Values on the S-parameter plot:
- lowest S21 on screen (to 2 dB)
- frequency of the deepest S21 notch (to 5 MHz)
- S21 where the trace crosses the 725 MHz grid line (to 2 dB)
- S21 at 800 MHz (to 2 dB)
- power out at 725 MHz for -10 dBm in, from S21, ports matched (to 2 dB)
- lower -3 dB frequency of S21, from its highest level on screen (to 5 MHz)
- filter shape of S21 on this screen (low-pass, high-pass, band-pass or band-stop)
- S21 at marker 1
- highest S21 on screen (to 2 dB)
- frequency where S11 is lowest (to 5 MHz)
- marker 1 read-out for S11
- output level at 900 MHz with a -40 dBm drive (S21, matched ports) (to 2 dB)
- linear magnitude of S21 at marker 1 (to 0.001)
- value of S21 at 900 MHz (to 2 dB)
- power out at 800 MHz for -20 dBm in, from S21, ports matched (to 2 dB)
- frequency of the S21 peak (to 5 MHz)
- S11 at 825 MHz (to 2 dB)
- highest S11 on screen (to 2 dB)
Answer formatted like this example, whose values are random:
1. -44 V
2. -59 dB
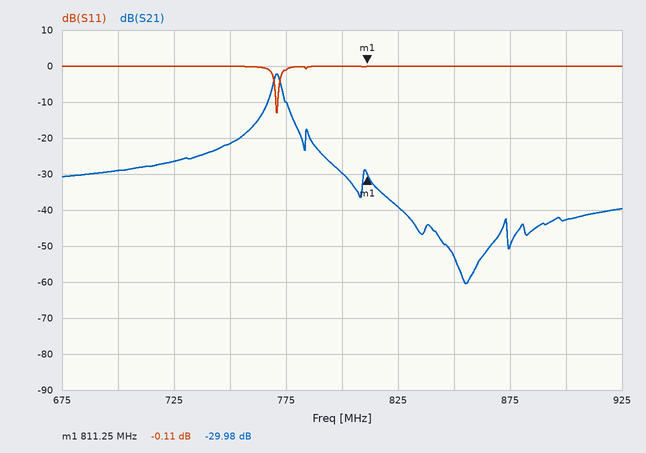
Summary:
1. -60 dB
2. 855 MHz
3. -26 dB
4. -30 dB
5. -36 dBm
6. 770 MHz
7. band-pass
8. -29.98 dB
9. -2 dB
10. 770 MHz
11. -0.11 dB
12. -82 dBm
13. 0.032
14. -42 dB
15. -50 dBm
16. 770 MHz
17. 0 dB
18. 0 dB
